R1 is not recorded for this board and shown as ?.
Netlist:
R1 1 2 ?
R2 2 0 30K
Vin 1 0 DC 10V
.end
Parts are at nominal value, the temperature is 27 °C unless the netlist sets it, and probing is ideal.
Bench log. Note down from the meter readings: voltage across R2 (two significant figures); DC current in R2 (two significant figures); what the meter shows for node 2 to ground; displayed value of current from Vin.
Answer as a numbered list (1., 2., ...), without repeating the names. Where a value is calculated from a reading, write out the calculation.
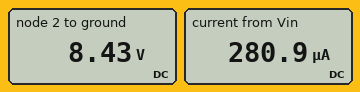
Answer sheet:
1. 8.43 V = 8.4 V
2. (8.43 V) / 30 kΩ = 280 µA
3. 8.43 V
4. 280.9 µA
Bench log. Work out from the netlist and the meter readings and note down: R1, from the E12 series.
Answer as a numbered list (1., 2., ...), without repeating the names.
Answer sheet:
1. 5.6 kΩ
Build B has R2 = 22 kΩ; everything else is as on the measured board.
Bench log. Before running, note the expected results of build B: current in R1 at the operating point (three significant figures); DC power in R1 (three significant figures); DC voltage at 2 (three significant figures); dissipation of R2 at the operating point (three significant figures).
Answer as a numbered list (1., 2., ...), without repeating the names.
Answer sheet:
1. 362 µA
2. 735 µW
3. 7.97 V
4. 2.89 mW
